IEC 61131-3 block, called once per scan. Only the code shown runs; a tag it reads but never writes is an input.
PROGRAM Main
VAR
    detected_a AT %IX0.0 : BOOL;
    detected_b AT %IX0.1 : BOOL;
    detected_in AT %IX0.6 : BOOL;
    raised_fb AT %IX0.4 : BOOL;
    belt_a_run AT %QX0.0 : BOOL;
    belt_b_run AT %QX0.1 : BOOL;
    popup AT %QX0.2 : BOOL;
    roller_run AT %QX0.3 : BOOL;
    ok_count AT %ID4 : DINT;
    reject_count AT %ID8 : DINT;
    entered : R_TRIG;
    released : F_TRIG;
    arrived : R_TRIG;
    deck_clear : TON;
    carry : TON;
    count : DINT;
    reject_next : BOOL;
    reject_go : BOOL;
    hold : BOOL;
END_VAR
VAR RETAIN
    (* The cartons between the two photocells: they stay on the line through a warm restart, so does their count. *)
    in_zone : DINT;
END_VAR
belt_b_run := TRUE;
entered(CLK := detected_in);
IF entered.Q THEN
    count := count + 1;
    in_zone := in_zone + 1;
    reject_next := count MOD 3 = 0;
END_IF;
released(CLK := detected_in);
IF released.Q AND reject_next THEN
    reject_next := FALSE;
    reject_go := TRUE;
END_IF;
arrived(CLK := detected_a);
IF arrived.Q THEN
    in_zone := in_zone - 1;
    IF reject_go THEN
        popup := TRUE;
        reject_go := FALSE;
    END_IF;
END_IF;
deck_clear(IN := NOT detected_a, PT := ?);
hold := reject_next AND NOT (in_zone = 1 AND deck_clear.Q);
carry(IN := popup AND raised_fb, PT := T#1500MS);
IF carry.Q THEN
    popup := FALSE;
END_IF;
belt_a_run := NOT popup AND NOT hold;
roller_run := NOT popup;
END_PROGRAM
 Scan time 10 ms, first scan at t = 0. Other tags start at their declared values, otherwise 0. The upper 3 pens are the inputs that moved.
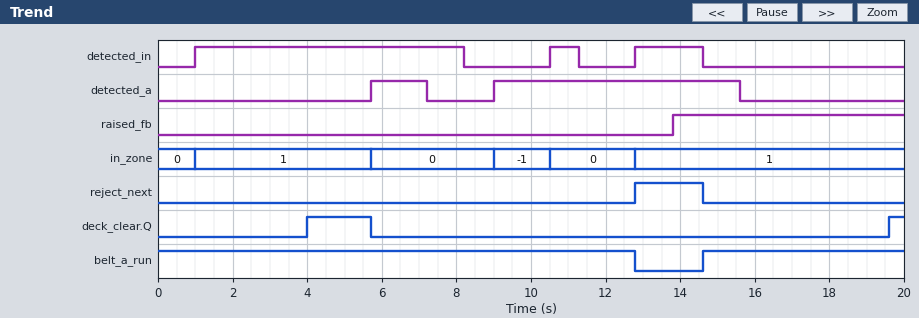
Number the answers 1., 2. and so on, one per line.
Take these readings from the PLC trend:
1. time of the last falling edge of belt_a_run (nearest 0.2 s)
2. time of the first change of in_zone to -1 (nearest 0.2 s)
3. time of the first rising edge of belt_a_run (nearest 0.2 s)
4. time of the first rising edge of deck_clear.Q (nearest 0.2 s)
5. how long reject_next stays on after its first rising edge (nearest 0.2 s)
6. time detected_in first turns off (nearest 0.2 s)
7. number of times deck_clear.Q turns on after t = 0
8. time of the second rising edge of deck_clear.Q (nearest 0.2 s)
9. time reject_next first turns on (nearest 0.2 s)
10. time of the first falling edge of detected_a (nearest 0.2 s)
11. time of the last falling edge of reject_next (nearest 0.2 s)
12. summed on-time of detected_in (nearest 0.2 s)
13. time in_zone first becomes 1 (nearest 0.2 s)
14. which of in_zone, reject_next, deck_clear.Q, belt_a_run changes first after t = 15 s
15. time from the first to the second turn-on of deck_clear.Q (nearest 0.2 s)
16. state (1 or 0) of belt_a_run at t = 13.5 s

1. 12.8 s
2. 9.0 s
3. 14.6 s
4. 4.0 s
5. 1.8 s
6. 8.2 s
7. 2
8. 19.6 s
9. 12.8 s
10. 7.2 s
11. 14.6 s
12. 9.8 s
13. 1.0 s
14. deck_clear.Q
15. 15.6 s
16. 0
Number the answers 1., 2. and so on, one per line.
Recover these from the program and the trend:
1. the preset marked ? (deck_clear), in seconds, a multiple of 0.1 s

1. 4.0 s
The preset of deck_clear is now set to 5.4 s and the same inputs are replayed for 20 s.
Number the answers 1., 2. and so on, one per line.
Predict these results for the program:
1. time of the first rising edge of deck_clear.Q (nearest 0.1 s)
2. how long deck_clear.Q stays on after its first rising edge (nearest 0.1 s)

1. 5.4 s
2. 0.3 s
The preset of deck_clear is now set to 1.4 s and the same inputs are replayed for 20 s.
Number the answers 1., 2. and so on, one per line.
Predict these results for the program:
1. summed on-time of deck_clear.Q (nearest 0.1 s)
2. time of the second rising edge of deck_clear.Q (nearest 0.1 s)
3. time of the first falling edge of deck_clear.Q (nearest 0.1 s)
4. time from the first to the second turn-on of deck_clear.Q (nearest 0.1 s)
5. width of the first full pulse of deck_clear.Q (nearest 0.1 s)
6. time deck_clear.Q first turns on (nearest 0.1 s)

1. 7.7 s
2. 8.6 s
3. 5.7 s
4. 7.2 s
5. 4.3 s
6. 1.4 s
